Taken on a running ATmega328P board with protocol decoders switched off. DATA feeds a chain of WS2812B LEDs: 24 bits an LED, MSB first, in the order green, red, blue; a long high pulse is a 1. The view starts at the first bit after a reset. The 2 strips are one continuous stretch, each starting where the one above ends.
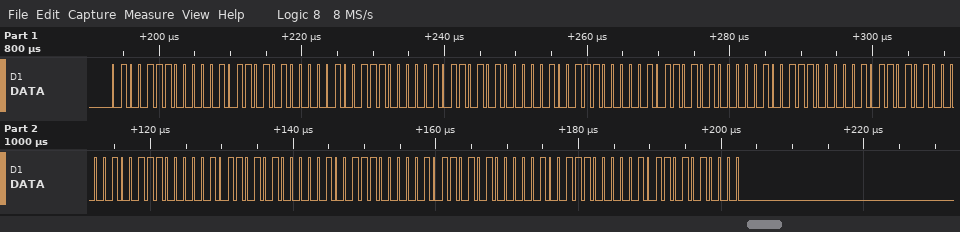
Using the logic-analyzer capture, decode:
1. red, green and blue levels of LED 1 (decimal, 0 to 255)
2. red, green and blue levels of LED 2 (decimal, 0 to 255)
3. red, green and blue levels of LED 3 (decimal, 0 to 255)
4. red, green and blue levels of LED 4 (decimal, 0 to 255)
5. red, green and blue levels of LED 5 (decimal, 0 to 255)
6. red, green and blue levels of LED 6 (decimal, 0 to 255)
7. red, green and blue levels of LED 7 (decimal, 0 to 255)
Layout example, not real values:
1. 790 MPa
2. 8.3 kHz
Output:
1. 11, 78, 80
2. 11, 78, 80
3. 11, 78, 80
4. 11, 78, 80
5. 11, 78, 80
6. 11, 78, 80
7. 11, 78, 80
